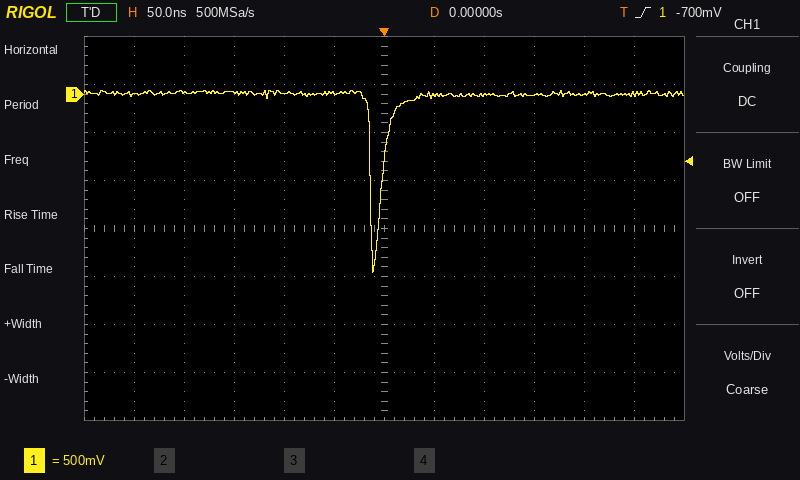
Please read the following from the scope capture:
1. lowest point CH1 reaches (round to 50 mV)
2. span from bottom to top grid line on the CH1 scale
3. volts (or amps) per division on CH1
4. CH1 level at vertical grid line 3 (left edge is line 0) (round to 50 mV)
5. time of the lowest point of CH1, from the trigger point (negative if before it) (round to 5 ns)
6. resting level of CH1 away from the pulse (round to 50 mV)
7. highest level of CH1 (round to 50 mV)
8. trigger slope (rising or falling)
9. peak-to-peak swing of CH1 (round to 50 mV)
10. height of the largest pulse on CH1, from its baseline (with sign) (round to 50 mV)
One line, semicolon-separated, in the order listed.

-1.85 V; 4 V; 500 mV; 0 mV; -10 ns; 0 mV; 50 mV; rising; 1.90 V; -1.85 V
